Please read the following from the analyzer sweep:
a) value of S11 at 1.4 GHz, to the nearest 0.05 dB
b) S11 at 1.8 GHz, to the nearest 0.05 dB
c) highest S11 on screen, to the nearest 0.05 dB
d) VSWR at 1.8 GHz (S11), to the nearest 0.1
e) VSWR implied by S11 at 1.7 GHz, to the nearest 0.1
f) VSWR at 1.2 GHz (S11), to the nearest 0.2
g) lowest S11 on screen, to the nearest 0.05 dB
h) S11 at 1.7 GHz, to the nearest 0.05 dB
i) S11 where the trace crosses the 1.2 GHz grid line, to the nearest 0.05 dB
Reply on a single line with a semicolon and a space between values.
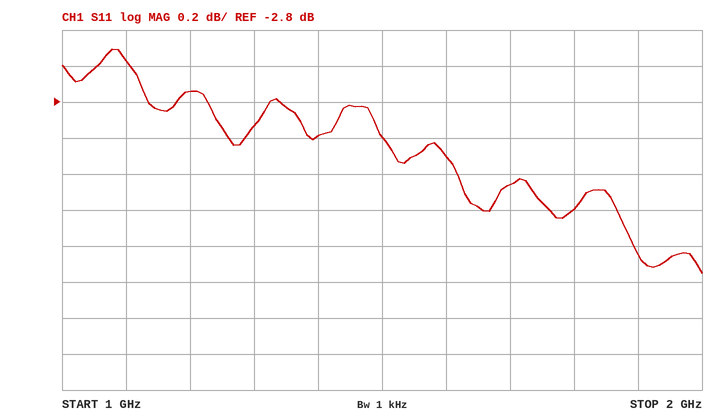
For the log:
-3.00 dB; -3.40 dB; -2.50 dB; 5.2; 5.4; 6.4; -3.75 dB; -3.25 dB; -2.75 dB
